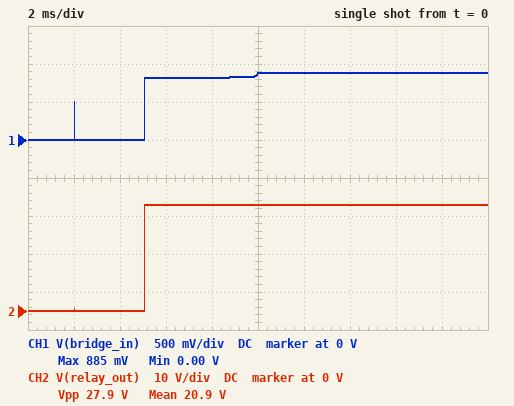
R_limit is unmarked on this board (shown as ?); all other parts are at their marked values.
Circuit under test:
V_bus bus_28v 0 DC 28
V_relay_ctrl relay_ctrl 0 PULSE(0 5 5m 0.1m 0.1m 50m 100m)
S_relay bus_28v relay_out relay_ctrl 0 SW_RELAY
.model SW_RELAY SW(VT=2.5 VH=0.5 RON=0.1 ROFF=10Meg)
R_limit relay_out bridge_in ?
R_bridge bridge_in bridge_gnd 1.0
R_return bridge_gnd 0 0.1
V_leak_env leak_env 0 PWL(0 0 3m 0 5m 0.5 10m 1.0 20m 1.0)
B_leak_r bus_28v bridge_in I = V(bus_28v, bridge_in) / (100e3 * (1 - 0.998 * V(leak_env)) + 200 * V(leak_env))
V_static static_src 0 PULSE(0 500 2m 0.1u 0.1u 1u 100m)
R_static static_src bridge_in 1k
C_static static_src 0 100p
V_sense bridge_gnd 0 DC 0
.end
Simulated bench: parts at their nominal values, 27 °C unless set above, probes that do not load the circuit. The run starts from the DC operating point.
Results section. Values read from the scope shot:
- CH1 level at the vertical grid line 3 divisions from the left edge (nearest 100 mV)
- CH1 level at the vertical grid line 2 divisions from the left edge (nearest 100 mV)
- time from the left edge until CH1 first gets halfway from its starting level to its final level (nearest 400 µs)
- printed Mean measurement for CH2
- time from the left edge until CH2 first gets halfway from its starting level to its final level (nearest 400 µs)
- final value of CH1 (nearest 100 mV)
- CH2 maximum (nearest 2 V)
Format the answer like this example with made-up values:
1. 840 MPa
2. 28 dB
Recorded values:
1. 800 mV
2. 0 V
3. 5.2 ms
4. 20.9 V
5. 5.2 ms
6. 900 mV
7. 28 V
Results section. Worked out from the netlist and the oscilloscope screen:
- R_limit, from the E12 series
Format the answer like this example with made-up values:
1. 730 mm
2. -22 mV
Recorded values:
1. 33 Ω
